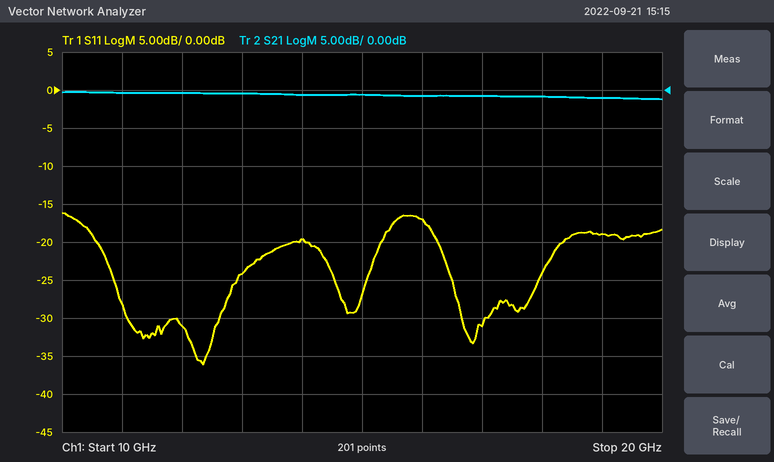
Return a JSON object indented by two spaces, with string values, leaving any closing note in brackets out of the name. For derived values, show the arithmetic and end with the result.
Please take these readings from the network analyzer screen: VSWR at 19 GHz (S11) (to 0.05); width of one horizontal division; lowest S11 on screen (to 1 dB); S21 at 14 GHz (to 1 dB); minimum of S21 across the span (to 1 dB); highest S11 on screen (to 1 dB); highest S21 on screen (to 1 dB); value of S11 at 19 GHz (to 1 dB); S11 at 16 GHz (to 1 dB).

{
  "VSWR at 19 GHz (S11)": "|Γ| = 10^(-19/20) = 0.1122; VSWR = (1 + 0.1122)/(1 − 0.1122) ≈ 1.25",
  "width of one horizontal division": "1 GHz",
  "lowest S11 on screen": "-36 dB",
  "S21 at 14 GHz": "-1 dB",
  "minimum of S21 across the span": "-1 dB",
  "highest S11 on screen": "-16 dB",
  "highest S21 on screen": "0 dB",
  "value of S11 at 19 GHz": "-19 dB",
  "S11 at 16 GHz": "-17 dB"
}
